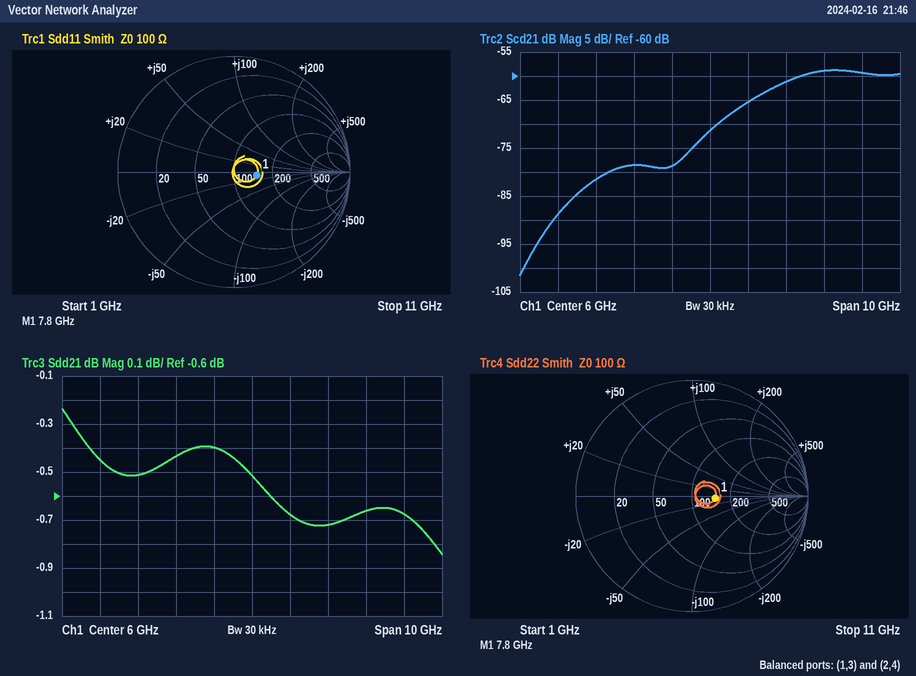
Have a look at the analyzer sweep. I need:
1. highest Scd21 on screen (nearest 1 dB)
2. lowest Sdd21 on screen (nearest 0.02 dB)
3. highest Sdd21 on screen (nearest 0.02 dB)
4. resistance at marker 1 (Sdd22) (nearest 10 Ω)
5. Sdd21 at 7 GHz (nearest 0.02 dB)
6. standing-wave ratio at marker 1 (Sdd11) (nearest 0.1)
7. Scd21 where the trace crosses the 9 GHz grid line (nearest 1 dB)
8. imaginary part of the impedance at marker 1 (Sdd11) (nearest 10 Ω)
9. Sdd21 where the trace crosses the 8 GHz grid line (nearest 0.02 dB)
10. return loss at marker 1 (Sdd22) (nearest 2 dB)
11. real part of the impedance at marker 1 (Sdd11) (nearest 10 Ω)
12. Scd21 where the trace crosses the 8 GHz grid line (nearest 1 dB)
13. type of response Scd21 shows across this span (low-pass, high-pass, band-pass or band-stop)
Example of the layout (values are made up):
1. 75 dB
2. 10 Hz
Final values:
1. -59 dB
2. -0.84 dB
3. -0.24 dB
4. 150 Ω
5. -0.68 dB
6. 1.5
7. -59 dB
8. -10 Ω
9. -0.72 dB
10. 14 dB
11. 150 Ω
12. -61 dB
13. high-pass
